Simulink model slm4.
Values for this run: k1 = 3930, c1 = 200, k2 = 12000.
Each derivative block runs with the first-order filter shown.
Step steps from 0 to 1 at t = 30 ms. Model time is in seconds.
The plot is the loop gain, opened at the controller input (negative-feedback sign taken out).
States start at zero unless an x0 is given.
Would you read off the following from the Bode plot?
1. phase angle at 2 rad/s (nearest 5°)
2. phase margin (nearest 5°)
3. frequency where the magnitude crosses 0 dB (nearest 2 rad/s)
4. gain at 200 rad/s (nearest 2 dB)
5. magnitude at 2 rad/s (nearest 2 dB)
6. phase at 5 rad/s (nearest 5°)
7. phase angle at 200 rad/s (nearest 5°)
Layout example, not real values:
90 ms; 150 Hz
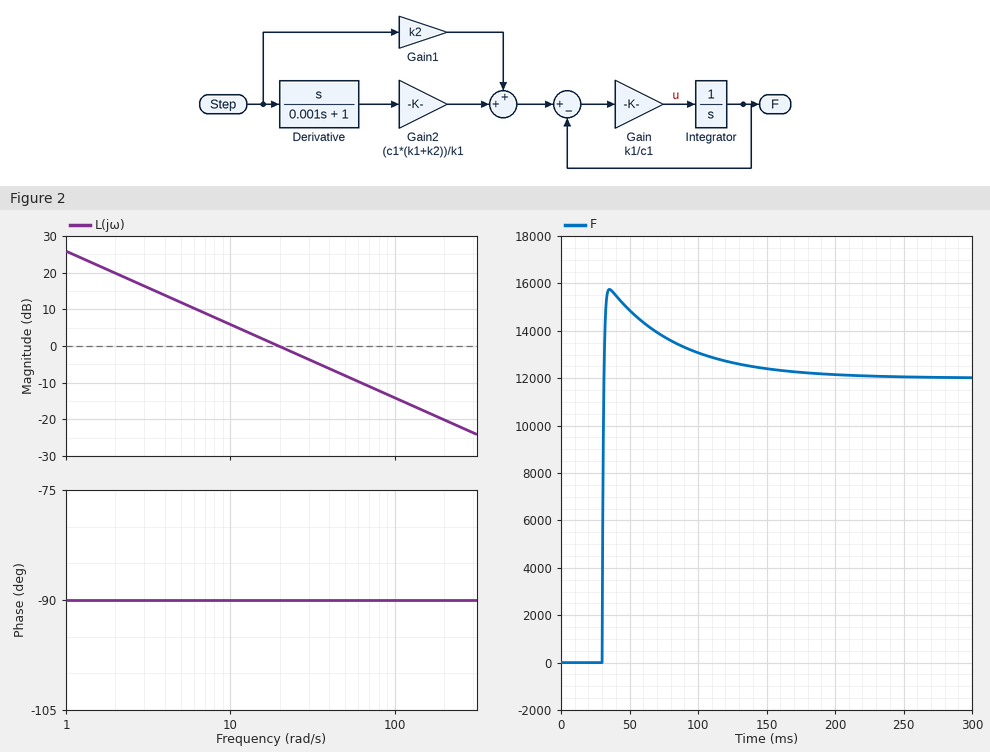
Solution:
-90°; 90°; 20 rad/s; -20 dB; 20 dB; -90°; -90°
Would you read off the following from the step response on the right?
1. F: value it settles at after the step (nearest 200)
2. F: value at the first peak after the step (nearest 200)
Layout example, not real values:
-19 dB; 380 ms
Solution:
12000; 15800
